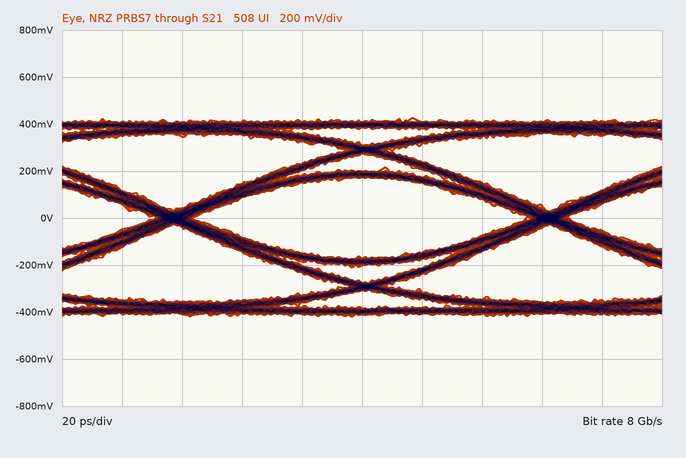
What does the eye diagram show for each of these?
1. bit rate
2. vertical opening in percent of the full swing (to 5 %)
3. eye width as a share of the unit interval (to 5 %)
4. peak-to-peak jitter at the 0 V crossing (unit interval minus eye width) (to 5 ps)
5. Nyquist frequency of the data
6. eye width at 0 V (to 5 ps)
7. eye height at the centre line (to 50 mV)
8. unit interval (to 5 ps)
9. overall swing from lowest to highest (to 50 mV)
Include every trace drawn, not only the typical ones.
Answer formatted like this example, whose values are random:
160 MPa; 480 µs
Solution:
8 Gb/s; 40 %; 90 %; 15 ps; 4 GHz; 110 ps; 350 mV; 125 ps; 850 mV
